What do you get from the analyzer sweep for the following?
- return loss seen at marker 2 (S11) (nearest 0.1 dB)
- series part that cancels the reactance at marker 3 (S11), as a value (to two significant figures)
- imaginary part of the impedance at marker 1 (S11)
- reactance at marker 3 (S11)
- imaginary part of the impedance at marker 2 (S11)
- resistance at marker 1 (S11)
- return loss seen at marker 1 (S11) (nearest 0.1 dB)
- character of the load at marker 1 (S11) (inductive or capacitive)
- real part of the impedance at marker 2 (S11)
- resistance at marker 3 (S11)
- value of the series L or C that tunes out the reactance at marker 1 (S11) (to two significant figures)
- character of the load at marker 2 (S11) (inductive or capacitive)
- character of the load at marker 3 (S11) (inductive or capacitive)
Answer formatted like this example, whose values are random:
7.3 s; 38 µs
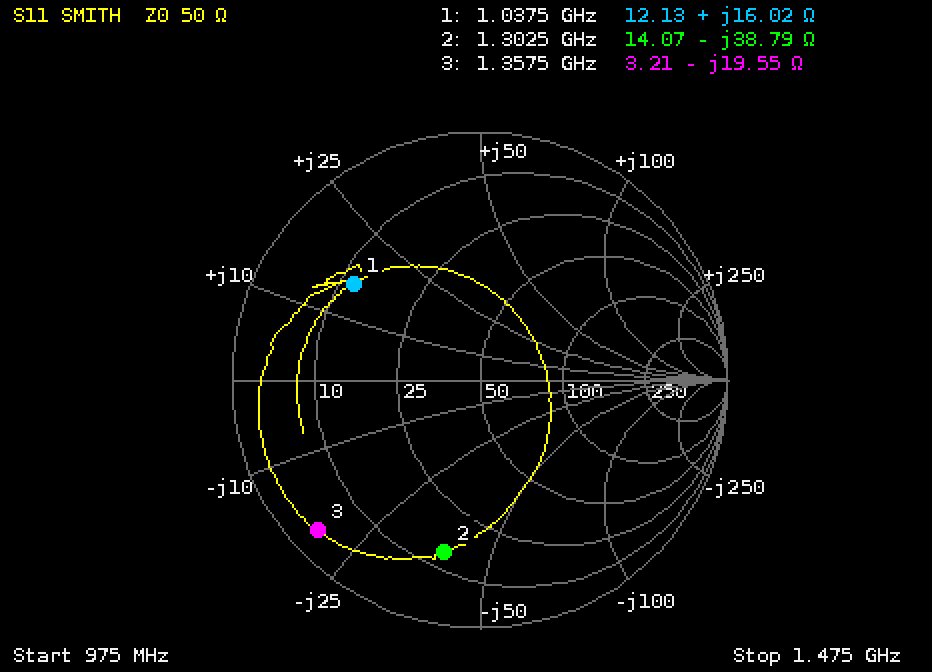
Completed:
3.0 dB; 2.3 nH; +16.02 Ω; -19.55 Ω; -38.79 Ω; 12.13 Ω; 3.9 dB; inductive; 14.07 Ω; 3.21 Ω; 9.6 pF; capacitive; capacitive
